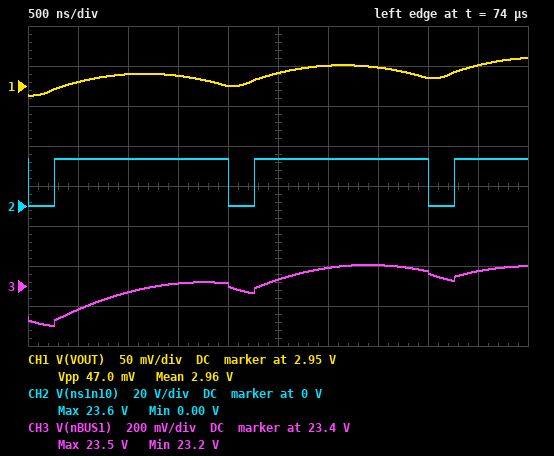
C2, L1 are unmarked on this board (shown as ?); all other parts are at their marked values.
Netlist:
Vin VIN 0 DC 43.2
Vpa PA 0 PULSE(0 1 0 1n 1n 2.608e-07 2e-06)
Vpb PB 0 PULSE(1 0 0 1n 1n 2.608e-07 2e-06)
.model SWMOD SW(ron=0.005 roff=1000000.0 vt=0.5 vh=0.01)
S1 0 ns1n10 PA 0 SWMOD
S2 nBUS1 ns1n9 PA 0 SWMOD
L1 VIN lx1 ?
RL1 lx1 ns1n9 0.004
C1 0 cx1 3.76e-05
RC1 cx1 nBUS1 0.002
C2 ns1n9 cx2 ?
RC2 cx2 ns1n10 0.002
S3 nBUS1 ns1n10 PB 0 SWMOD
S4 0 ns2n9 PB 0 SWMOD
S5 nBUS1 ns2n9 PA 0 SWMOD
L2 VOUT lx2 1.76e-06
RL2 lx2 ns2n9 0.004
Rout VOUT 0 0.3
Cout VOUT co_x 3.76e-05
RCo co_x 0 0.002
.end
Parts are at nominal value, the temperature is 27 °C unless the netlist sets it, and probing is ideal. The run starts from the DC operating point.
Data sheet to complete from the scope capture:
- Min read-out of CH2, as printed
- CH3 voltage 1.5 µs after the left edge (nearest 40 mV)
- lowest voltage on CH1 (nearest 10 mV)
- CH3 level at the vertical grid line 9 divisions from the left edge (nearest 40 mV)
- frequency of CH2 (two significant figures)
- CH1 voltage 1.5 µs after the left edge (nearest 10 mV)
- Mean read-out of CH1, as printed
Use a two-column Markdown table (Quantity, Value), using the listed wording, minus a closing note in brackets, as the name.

| Quantity | Value |
|---|---|
| Min read-out of CH2, as printed | 0.00 V |
| CH3 voltage 1.5 µs after the left edge | 23.40 V |
| lowest voltage on CH1 | 2.94 V |
| CH3 level at the vertical grid line 9 divisions from the left edge | 23.48 V |
| frequency of CH2 | 500 kHz |
| CH1 voltage 1.5 µs after the left edge | 2.96 V |
| Mean read-out of CH1, as printed | 2.96 V |
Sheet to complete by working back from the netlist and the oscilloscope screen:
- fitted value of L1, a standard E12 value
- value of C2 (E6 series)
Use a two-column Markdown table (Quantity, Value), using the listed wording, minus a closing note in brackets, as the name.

| Quantity | Value |
|---|---|
| fitted value of L1, a standard E12 value | 560 nH |
| value of C2 | 47 µF |
